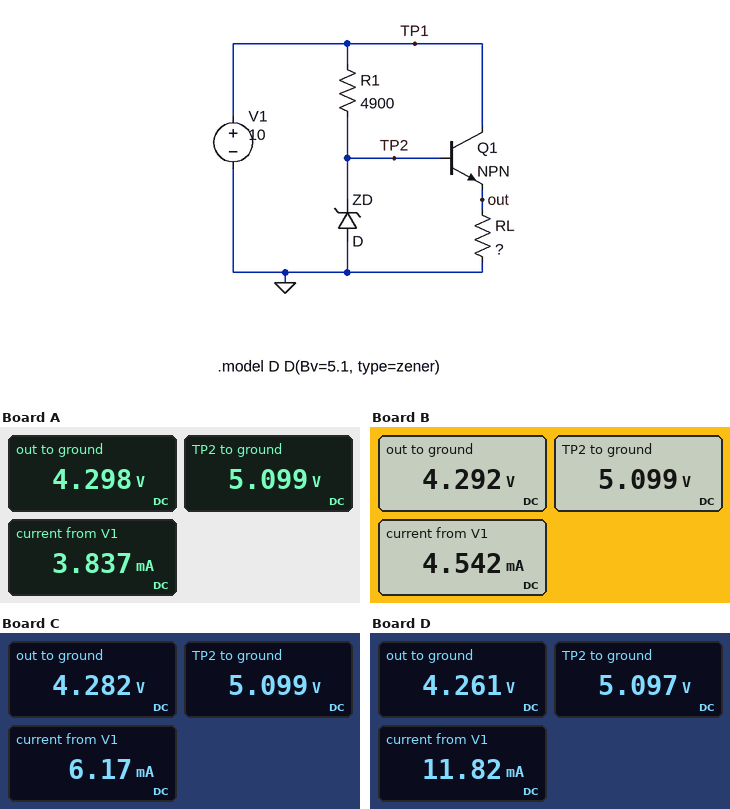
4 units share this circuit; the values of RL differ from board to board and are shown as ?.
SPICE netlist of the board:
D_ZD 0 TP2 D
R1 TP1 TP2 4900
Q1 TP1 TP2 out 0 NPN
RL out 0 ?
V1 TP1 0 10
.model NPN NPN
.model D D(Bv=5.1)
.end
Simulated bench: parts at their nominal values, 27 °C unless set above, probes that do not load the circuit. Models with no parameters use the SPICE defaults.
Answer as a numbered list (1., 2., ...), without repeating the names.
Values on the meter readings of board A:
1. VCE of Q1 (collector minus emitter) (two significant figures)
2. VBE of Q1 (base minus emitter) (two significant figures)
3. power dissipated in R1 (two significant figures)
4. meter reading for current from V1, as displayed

1. 5.7 V
2. 800 mV
3. 4.9 mW
4. 3.837 mA
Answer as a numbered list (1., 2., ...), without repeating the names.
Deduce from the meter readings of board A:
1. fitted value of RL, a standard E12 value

1. 1.5 kΩ
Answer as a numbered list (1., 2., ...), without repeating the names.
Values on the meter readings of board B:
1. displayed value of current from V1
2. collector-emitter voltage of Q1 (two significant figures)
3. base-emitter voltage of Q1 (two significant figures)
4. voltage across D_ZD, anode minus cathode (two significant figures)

1. 4.542 mA
2. 5.7 V
3. 810 mV
4. -5.1 V
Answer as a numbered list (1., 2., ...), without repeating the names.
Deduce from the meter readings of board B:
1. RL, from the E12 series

1. 1.2 kΩ
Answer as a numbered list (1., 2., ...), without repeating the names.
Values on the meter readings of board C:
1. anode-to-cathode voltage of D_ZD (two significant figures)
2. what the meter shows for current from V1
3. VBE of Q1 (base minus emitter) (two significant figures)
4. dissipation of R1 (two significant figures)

1. -5.1 V
2. 6.17 mA
3. 820 mV
4. 4.9 mW
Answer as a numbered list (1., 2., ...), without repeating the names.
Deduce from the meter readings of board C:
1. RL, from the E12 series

1. 820 Ω
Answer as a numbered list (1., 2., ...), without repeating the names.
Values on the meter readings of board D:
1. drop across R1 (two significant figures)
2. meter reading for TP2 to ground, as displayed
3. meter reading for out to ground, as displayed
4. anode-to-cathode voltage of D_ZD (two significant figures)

1. 4.9 V
2. 5.097 V
3. 4.261 V
4. -5.1 V
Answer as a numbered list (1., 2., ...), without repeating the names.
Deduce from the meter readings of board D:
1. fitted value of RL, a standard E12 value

1. 390 Ω
